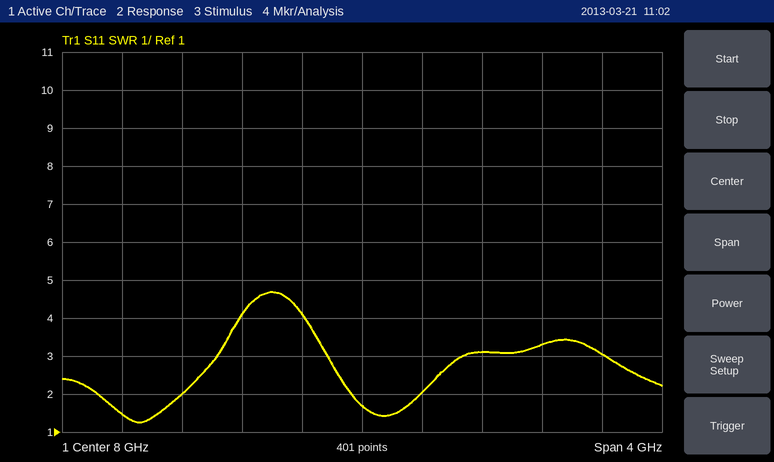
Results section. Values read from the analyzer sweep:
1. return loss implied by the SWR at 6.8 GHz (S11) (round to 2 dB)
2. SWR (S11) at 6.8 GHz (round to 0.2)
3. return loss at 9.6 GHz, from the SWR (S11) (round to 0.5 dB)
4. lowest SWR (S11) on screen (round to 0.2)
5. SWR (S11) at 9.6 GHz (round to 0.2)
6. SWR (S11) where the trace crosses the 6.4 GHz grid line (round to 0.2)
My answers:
10 dB
2.0
6.0 dB
1.2
3.0
1.4
